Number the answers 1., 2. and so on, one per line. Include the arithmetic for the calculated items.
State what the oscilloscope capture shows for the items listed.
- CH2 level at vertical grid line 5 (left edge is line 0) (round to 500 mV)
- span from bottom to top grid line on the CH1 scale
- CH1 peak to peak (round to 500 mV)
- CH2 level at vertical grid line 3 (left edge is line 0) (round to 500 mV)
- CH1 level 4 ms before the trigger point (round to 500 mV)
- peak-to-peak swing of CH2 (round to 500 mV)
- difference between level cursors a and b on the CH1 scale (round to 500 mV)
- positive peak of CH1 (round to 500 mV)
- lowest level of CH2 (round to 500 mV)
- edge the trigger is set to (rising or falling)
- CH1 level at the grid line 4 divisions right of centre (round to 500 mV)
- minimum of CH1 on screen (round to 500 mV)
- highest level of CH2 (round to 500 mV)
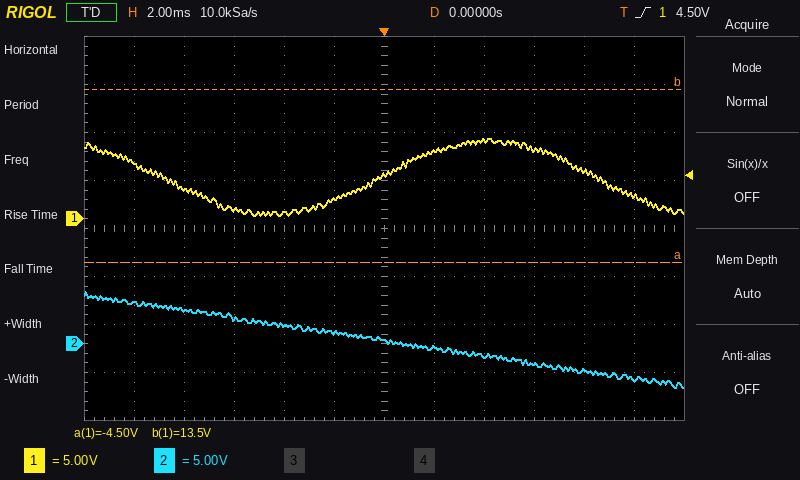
1. 1.0 V
2. 40 V
3. 8.5 V − (500 mV) = 8.0 V
4. 2.5 V
5. 500 mV
6. 5.5 V − (-4.5 V) = 10.0 V
7. 18.0 V
8. 8.5 V
9. -4.5 V
10. rising
11. 5.0 V
12. 500 mV
13. 5.5 V
